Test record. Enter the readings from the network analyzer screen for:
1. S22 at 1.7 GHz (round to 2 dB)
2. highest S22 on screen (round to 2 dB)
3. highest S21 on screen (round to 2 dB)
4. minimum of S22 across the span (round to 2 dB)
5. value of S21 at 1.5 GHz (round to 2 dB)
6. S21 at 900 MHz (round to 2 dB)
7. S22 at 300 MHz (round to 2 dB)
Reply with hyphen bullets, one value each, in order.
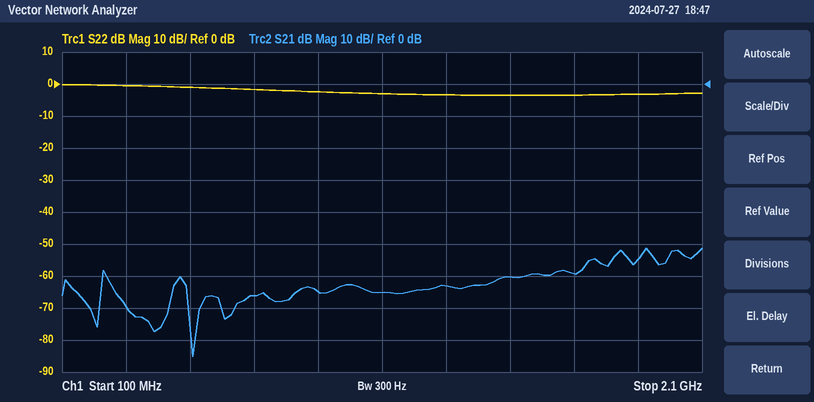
- -4 dB
- 0 dB
- -52 dB
- -4 dB
- -60 dB
- -64 dB
- 0 dB
